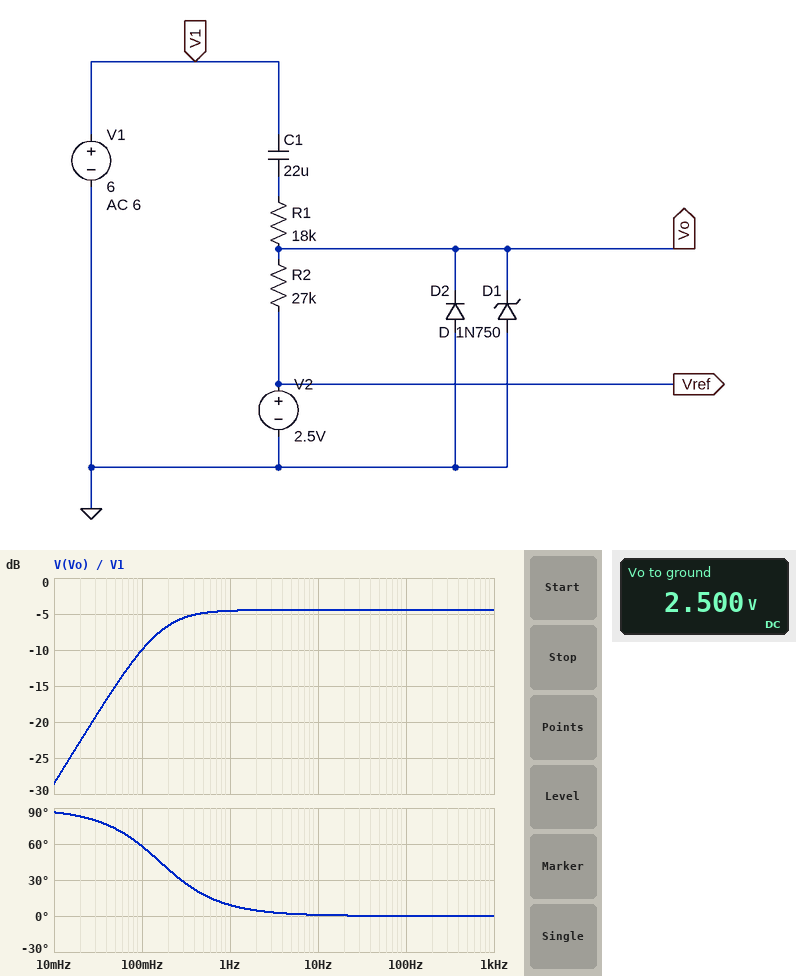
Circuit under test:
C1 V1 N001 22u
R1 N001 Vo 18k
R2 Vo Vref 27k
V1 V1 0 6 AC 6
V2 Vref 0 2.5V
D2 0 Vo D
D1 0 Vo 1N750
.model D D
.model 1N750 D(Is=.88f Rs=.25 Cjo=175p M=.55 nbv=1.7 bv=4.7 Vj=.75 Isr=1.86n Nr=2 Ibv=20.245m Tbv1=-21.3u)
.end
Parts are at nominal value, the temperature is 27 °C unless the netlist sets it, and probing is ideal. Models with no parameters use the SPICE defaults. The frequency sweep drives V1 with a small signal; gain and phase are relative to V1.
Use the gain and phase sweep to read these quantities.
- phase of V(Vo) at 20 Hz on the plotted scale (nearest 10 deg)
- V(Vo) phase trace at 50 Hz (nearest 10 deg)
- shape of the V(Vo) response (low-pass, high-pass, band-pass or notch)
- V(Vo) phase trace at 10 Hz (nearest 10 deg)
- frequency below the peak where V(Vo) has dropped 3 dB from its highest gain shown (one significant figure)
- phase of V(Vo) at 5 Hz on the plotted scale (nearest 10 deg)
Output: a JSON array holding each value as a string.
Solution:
["0 deg", "0 deg", "high-pass", "0 deg", "200 mHz", "0 deg"]
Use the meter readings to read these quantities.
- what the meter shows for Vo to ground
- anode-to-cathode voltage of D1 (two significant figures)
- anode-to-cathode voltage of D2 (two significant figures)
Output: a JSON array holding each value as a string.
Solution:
["2.500 V", "-2.5 V", "-2.5 V"]
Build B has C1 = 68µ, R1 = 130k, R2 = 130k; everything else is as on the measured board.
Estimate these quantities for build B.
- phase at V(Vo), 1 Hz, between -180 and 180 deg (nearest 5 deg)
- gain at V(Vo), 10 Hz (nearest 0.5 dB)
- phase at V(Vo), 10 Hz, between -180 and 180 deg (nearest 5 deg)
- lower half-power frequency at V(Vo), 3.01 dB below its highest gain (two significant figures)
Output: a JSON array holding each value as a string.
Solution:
["0 deg", "-6.0 dB", "0 deg", "9.0 mHz"]
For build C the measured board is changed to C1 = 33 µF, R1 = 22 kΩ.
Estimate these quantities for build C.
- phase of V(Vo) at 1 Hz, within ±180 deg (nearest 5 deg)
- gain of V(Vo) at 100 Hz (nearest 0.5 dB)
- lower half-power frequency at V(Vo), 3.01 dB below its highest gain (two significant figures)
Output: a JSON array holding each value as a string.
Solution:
["5 deg", "-5.0 dB", "98 mHz"]
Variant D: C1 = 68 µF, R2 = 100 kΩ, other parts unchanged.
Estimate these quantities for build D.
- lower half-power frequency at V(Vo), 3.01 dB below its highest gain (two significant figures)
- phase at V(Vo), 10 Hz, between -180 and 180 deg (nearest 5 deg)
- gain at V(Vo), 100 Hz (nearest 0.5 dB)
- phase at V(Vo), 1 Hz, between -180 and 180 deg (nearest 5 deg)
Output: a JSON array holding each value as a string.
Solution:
["20 mHz", "0 deg", "-1.5 dB", "0 deg"]
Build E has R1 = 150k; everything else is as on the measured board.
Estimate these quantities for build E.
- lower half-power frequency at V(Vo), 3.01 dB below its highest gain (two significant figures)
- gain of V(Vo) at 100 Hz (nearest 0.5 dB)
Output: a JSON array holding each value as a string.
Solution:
["41 mHz", "-16.5 dB"]
